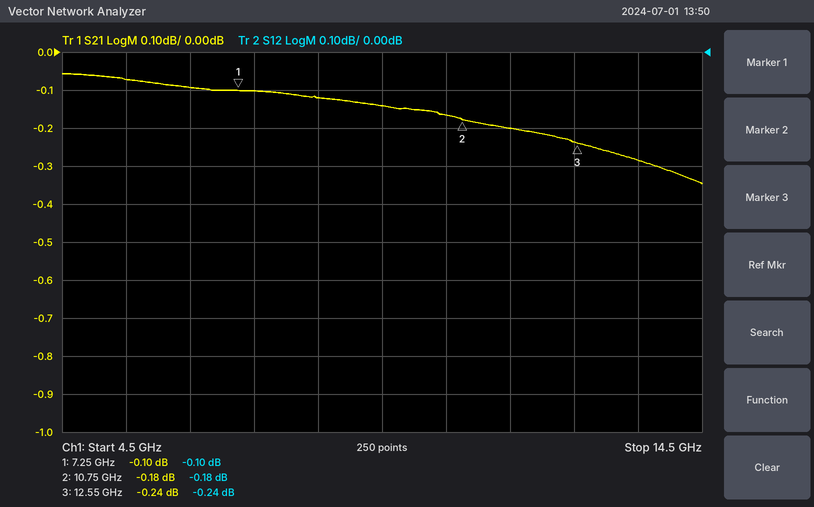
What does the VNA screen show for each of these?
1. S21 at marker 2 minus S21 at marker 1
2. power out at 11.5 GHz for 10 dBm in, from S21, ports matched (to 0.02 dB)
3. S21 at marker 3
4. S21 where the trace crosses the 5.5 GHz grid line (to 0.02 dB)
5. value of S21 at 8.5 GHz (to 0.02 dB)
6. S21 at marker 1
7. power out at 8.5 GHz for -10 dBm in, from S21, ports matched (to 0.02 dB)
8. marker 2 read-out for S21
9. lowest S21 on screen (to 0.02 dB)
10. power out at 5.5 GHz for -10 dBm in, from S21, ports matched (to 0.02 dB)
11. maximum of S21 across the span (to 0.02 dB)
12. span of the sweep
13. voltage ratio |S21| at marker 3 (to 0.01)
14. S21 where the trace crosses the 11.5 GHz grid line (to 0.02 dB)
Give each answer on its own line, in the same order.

-0.08 dB
9.80 dBm
-0.24 dB
-0.08 dB
-0.12 dB
-0.10 dB
-10.12 dBm
-0.18 dB
-0.34 dB
-10.08 dBm
-0.06 dB
10 GHz
0.97
-0.20 dB
